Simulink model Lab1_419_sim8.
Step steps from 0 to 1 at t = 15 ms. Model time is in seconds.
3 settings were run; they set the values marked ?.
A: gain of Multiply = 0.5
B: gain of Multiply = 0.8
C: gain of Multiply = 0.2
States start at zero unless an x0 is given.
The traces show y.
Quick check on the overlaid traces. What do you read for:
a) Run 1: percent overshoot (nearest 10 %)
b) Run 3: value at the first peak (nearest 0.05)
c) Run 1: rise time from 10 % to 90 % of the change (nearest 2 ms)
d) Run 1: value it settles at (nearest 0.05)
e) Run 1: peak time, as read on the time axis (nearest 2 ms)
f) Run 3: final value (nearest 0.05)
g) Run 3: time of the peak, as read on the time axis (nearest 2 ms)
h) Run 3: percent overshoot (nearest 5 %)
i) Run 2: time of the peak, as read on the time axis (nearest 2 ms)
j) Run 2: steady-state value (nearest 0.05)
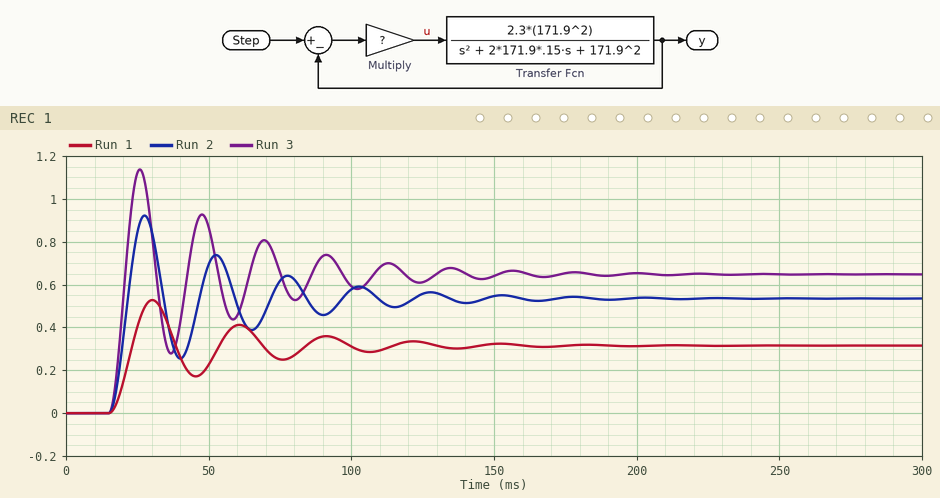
70 %
1.15
6 ms
0.30
30 ms
0.65
26 ms
75 %
28 ms
0.55
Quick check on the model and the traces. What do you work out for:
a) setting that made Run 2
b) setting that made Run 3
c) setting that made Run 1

A
B
C
